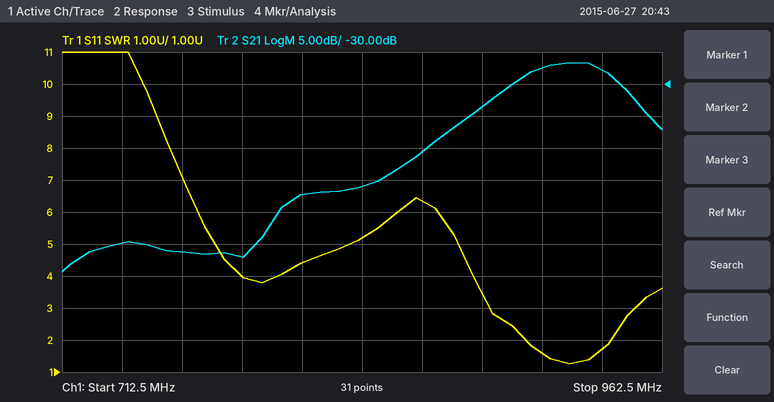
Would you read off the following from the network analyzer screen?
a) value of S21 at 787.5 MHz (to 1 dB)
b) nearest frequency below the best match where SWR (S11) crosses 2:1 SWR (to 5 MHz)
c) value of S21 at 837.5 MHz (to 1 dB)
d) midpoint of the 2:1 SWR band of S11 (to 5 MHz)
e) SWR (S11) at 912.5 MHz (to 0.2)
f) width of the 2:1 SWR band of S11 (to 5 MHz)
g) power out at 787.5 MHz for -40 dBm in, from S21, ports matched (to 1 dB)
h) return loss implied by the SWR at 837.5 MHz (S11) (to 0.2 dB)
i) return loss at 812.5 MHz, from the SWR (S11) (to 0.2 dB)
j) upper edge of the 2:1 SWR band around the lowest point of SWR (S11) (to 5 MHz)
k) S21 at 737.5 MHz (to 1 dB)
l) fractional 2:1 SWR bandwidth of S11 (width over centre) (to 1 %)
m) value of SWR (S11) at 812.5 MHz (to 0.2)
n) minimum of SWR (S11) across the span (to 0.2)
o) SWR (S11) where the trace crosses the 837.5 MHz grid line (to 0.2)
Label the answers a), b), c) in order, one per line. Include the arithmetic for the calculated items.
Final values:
a) -57 dB
b) 905 MHz
c) -46 dB
d) 925 MHz
e) 1.6
f) 940 MHz − 905 MHz = 35 MHz
g) -40 dBm + (-57 dB) = -97 dBm
h) −20 log10((5.2 − 1)/(5.2 + 1)) ≈ 3.4 dB
i) −20 log10((4.4 − 1)/(4.4 + 1)) ≈ 4.0 dB
j) 940 MHz
k) -55 dB
l) 35 MHz / 922.5 MHz ≈ 4 %
m) 4.4
n) 1.2
o) 5.2
